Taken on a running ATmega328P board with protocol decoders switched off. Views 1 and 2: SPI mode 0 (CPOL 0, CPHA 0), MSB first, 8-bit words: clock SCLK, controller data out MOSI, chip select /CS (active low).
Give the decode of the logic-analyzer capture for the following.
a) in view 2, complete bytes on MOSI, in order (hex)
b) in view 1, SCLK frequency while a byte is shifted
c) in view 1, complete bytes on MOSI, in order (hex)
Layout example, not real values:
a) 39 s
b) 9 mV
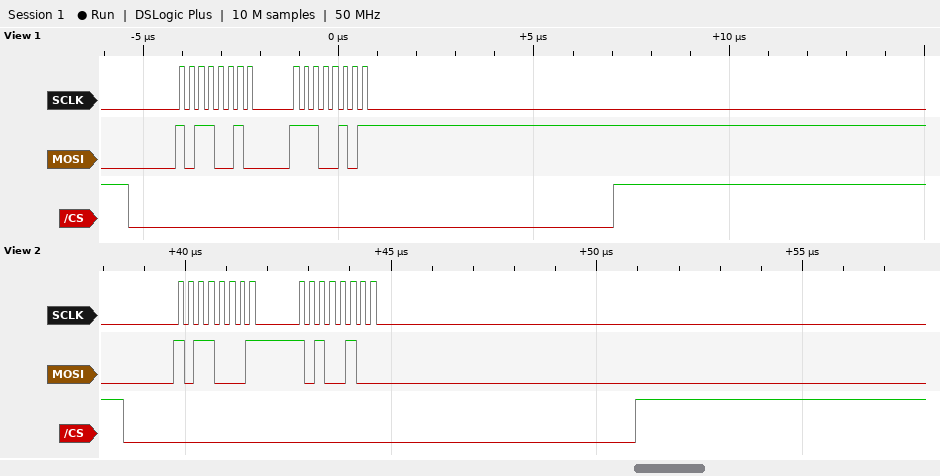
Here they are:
a) B1 A4
b) 4 MHz
c) B2 E5
